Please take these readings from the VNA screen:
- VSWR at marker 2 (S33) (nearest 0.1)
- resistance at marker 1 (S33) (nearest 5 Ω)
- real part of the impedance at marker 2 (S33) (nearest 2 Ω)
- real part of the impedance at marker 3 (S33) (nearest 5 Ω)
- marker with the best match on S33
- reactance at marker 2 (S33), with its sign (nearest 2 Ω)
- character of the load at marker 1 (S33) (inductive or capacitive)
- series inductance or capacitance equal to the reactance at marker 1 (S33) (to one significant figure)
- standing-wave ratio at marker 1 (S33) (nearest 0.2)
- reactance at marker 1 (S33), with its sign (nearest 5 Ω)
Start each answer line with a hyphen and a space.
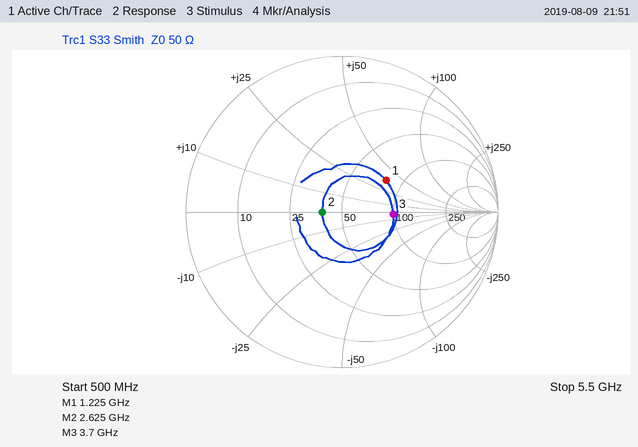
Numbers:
- 1.3
- 80 Ω
- 38 Ω
- 100 Ω
- marker 2
- 0 Ω
- inductive
- 5 nH
- 2.0
- +35 Ω
